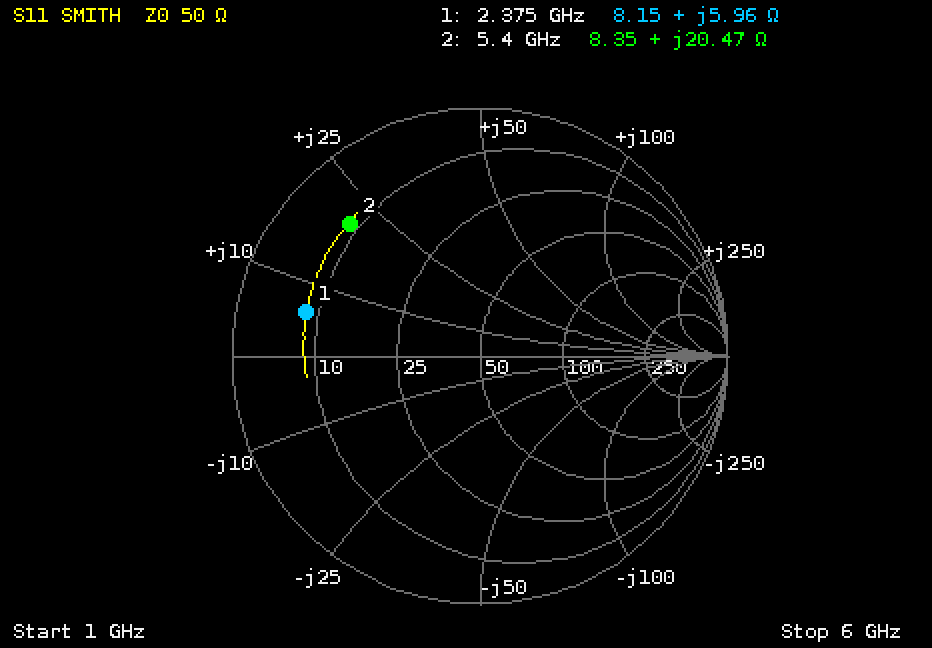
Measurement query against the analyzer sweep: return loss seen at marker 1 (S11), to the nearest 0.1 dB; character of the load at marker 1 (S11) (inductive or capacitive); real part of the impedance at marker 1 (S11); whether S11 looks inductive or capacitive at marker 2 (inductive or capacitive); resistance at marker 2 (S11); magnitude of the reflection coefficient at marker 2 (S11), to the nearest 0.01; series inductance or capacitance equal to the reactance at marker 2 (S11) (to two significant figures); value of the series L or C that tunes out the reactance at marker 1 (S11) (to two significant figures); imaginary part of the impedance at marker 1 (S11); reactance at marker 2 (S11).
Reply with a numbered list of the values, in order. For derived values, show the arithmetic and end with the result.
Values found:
1. 2.8 dB
2. inductive
3. 8.15 Ω
4. inductive
5. 8.35 Ω
6. 0.75
7. L = 20.47 Ω/(2π × 5.4 GHz) ≈ 603 pH, so 600 pH to two significant figures
8. C = 1/(2π × 2.375 GHz × 5.96 Ω) ≈ 11 pF
9. +5.96 Ω
10. +20.47 Ω
